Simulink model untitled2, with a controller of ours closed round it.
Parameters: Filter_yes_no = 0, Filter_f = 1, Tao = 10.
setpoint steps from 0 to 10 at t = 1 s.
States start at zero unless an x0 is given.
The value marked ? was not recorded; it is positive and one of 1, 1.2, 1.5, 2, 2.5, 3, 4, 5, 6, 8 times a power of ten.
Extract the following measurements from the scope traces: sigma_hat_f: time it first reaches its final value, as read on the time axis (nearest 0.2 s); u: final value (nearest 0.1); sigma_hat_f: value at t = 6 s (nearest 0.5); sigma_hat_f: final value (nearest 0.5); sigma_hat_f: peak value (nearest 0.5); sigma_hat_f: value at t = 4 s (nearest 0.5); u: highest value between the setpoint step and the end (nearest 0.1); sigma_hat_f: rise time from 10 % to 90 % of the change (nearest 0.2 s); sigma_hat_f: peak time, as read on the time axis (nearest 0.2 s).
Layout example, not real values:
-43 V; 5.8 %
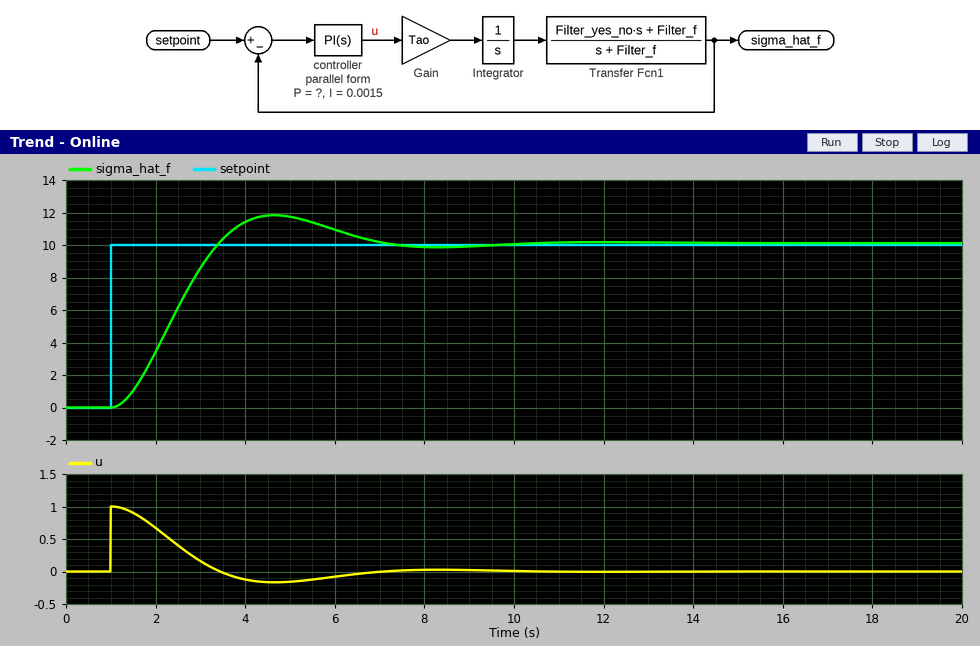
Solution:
3.4 s; 0.0; 11.0; 10.0; 12.0; 11.5; 1.0; 1.6 s; 4.6 s
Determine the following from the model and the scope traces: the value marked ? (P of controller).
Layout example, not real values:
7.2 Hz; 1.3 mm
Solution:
0.1
